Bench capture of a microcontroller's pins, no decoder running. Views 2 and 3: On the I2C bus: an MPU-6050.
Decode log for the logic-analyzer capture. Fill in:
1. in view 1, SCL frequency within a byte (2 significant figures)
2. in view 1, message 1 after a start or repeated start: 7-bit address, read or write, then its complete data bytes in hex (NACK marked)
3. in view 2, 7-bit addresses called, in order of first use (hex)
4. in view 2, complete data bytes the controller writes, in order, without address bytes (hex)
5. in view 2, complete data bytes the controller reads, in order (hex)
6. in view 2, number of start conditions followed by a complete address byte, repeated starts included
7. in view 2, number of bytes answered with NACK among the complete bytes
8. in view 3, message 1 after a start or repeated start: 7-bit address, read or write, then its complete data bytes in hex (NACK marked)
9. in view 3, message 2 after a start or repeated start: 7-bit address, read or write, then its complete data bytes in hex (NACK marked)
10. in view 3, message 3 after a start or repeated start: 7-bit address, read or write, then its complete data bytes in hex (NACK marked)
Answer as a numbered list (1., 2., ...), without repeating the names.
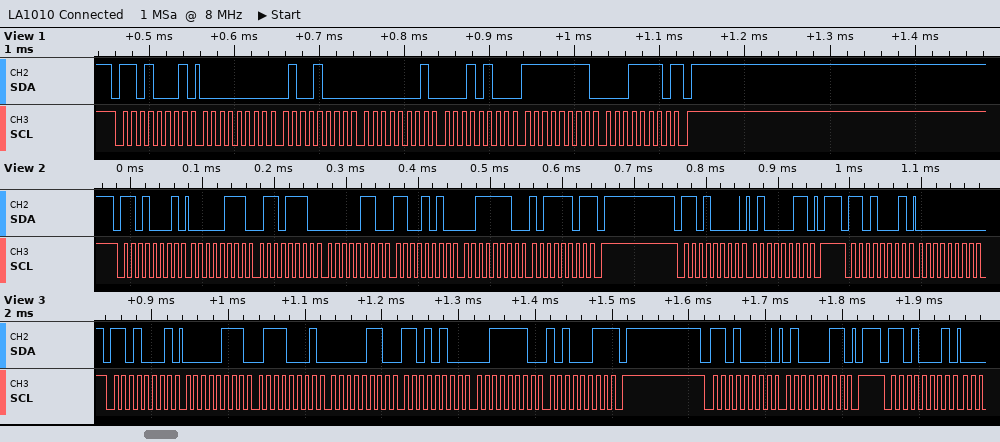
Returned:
1. 100 kHz
2. 0x68 read: 00 48 01 14 FF 1E NACK
3. 0x68
4. 43
5. 07 6E 06 CA 3E BD 00
6. 3
7. 1
8. 0x68 read: 07 71 06 D4 3E A3 NACK
9. 0x68 write: 43
10. 0x68 read
